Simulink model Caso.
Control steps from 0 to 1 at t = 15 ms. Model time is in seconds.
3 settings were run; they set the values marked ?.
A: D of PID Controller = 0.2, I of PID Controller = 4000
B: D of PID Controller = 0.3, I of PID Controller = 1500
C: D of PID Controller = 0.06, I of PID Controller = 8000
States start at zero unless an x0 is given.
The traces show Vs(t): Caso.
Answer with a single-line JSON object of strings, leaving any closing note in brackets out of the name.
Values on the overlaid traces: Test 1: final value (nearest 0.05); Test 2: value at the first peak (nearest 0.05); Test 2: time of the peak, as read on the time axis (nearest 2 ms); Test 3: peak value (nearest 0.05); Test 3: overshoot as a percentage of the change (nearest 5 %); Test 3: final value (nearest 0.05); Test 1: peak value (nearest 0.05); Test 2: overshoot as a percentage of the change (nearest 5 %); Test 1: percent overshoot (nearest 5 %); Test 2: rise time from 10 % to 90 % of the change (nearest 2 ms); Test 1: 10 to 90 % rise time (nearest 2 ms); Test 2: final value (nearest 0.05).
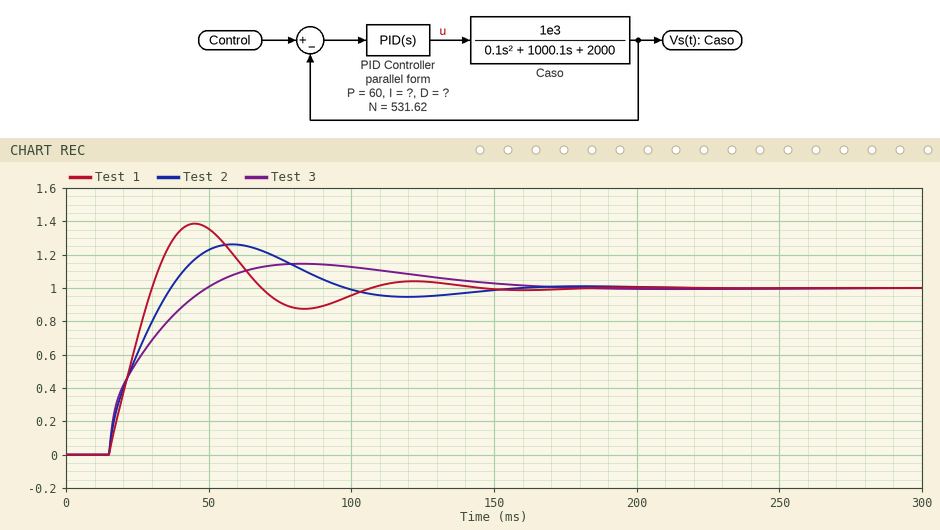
{"Test 1: final value": "1.00", "Test 2: value at the first peak": "1.25", "Test 2: time of the peak, as read on the time axis": "58 ms", "Test 3: peak value": "1.15", "Test 3: overshoot as a percentage of the change": "15 %", "Test 3: final value": "1.00", "Test 1: peak value": "1.40", "Test 2: overshoot as a percentage of the change": "25 %", "Test 1: percent overshoot": "40 %", "Test 2: rise time from 10 % to 90 % of the change": "18 ms", "Test 1: 10 to 90 % rise time": "12 ms", "Test 2: final value": "1.00"}
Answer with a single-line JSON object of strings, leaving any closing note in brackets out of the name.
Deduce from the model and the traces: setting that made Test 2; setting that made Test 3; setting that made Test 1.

{"setting that made Test 2": "A", "setting that made Test 3": "B", "setting that made Test 1": "C"}
